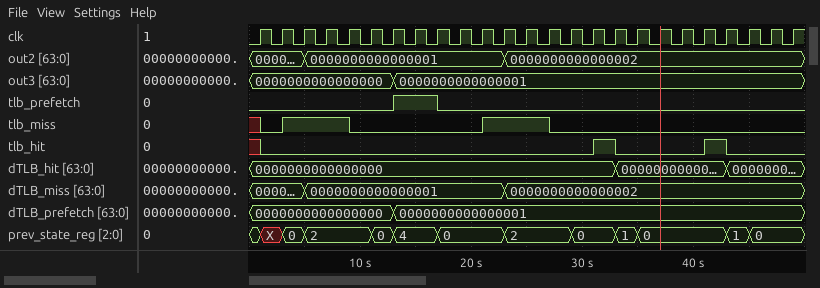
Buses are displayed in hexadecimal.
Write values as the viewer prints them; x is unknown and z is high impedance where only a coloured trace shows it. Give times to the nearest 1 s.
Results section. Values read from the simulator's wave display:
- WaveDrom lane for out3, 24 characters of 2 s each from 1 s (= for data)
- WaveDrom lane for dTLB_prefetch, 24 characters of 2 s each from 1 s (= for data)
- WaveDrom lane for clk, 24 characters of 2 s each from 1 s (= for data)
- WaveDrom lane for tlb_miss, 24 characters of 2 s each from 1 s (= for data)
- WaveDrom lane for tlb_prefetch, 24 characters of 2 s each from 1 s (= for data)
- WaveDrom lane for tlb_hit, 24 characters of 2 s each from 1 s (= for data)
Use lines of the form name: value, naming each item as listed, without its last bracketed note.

WaveDrom lane for out3, 24 characters of 2 s each from 1 s: {name: 'out3', wave: '=.....=.................', data: '0000000000000000 0000000000000001'}
WaveDrom lane for dTLB_prefetch, 24 characters of 2 s each from 1 s: {name: 'dTLB_prefetch', wave: '=.....=.................', data: '0000000000000000 0000000000000001'}
WaveDrom lane for clk, 24 characters of 2 s each from 1 s: {name: 'clk', wave: 'p.......................'}
WaveDrom lane for tlb_miss, 24 characters of 2 s each from 1 s: {name: 'tlb_miss', wave: '01..0.....1..0..........'}
WaveDrom lane for tlb_prefetch, 24 characters of 2 s each from 1 s: {name: 'tlb_prefetch', wave: '0.....1.0...............'}
WaveDrom lane for tlb_hit, 24 characters of 2 s each from 1 s: {name: 'tlb_hit', wave: '0..............10...10..'}
